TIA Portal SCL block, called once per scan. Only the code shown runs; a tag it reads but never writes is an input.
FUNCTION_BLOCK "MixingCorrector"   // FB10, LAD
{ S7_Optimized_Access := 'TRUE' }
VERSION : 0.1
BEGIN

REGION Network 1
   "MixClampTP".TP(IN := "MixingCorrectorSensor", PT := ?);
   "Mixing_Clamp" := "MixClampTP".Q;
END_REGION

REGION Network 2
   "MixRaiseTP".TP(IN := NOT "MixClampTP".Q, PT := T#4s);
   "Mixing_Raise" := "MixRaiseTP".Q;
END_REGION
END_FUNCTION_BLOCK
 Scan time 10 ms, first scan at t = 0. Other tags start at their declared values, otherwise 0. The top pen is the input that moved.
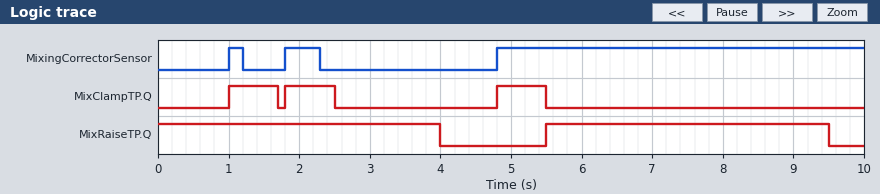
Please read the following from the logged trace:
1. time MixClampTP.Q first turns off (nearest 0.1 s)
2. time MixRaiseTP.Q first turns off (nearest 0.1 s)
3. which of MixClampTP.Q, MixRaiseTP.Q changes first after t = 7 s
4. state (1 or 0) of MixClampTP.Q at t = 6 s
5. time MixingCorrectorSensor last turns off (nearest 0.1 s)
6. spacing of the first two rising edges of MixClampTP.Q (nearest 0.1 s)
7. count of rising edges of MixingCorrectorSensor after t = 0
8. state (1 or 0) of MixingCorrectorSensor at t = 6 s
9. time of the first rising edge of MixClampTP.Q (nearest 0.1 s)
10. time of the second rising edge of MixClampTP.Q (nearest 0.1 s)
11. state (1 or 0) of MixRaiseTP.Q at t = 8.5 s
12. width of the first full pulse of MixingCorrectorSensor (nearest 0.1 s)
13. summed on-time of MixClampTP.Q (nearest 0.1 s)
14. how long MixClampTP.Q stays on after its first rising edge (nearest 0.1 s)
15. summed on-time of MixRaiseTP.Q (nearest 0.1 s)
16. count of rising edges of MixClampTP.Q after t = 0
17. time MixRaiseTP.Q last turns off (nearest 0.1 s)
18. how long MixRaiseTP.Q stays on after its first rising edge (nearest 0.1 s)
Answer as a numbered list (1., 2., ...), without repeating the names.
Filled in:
1. 1.7 s
2. 4.0 s
3. MixRaiseTP.Q
4. 0
5. 2.3 s
6. 0.8 s
7. 3
8. 1
9. 1.0 s
10. 1.8 s
11. 1
12. 0.2 s
13. 2.1 s
14. 0.7 s
15. 8.0 s
16. 3
17. 9.5 s
18. 4.0 s
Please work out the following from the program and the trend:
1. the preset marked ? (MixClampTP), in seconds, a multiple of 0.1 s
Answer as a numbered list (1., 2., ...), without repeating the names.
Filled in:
1. 0.7 s
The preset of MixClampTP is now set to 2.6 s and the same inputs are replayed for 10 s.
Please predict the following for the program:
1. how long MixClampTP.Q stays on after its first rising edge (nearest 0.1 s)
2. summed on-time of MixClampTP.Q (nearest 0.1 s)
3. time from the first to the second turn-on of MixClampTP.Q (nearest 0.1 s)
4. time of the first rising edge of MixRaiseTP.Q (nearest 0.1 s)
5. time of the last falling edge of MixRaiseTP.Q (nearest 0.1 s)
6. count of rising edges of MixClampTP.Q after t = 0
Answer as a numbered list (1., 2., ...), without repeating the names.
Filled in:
1. 2.6 s
2. 5.2 s
3. 3.8 s
4. 7.4 s
5. 4.0 s
6. 2
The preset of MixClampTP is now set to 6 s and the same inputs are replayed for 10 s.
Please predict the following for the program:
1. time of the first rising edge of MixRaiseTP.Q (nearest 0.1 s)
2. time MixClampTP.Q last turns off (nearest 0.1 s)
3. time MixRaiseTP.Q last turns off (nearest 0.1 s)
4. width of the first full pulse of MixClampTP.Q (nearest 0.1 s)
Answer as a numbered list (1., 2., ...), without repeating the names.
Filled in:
1. 7.0 s
2. 7.0 s
3. 4.0 s
4. 6.0 s
